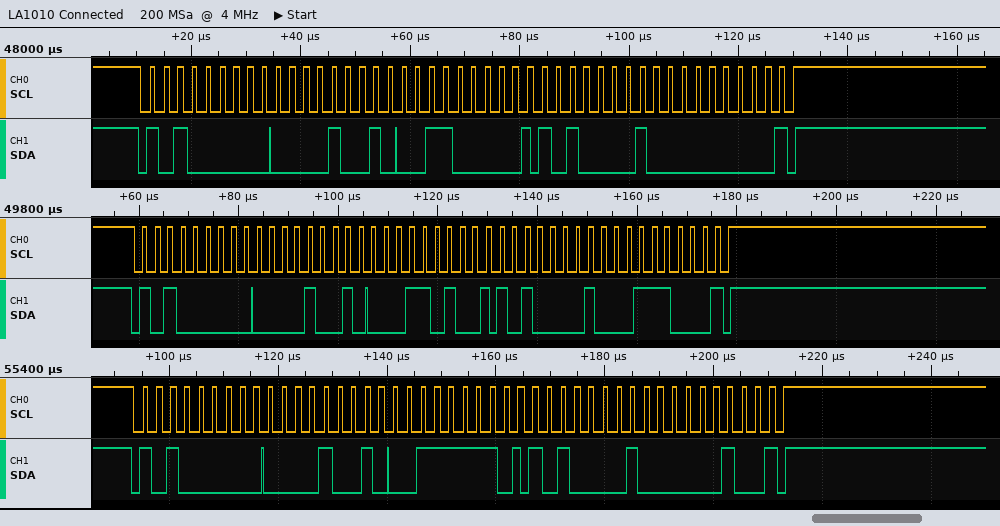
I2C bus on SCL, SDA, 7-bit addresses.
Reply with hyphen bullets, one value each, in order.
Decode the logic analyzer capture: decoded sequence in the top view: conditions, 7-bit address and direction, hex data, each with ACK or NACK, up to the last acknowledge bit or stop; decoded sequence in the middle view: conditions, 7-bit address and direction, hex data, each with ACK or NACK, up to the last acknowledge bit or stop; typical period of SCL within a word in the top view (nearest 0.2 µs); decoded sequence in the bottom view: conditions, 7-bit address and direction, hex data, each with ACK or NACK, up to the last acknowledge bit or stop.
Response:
- start, address 50 write ACK, 09 ACK, 30 ACK, repeated start, address 50 read ACK, 00 NACK, stop
- start, address 50 write ACK, 09 ACK, 1A ACK, repeated start, address 50 read ACK, 38 NACK, stop
- 2.6 µs
- start, address 50 write ACK, 09 ACK, 3F ACK, repeated start, address 50 read ACK, 04 NACK, stop
